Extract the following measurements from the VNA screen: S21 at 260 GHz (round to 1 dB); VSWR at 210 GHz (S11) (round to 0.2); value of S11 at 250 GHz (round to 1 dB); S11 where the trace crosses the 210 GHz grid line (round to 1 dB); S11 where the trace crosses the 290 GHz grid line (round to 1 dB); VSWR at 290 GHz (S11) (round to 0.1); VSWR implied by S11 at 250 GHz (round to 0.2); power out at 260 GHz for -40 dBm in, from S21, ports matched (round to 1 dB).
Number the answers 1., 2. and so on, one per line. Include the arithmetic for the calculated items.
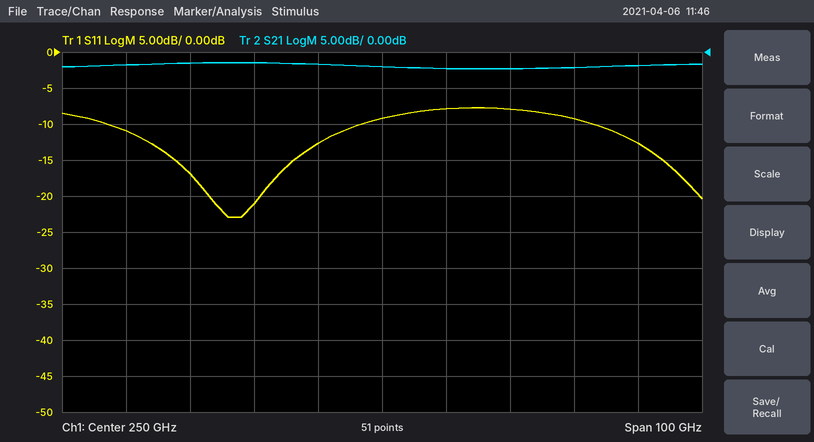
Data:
1. -2 dB
2. |Γ| = 10^(-11/20) = 0.2818; VSWR = (1 + 0.2818)/(1 − 0.2818) ≈ 1.8
3. -9 dB
4. -11 dB
5. -13 dB
6. |Γ| = 10^(-13/20) = 0.2239; VSWR = (1 + 0.2239)/(1 − 0.2239) ≈ 1.6
7. |Γ| = 10^(-9/20) = 0.3548; VSWR = (1 + 0.3548)/(1 − 0.3548) ≈ 2.10, so 2.0 to the nearest 0.2
8. -40 dBm + (-2 dB) = -42 dBm
